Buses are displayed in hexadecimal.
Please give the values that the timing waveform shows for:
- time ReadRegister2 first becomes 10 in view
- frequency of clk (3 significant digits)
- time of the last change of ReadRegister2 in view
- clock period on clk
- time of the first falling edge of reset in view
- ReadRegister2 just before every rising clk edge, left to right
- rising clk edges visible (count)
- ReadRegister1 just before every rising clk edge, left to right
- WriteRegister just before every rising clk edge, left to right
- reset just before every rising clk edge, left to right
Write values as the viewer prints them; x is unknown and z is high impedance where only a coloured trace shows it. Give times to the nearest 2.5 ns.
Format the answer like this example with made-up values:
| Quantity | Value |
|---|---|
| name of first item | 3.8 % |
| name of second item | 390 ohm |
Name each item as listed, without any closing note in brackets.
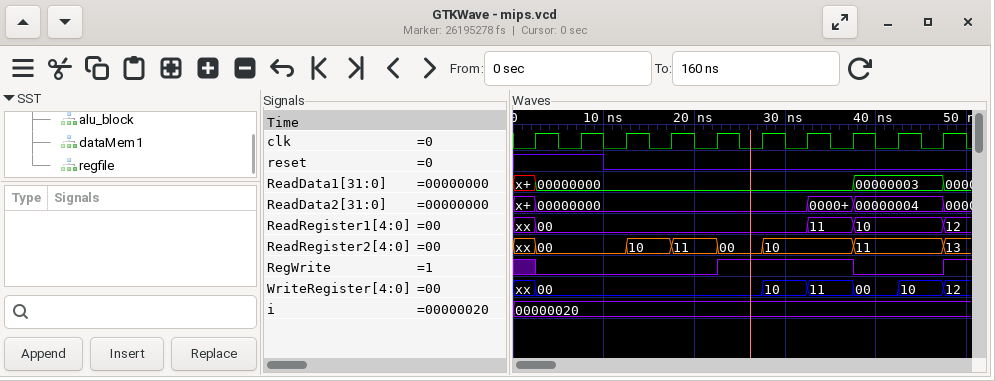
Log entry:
| Quantity | Value |
|---|---|
| time ReadRegister2 first becomes 10 in view | 12.5 ns |
| frequency of clk | 200 MHz |
| time of the last change of ReadRegister2 in view | 47.5 ns |
| clock period on clk | 5 ns |
| time of the first falling edge of reset in view | 10 ns |
| ReadRegister2 just before every rising clk edge, left to right | xx, 00, 00, 10, 11, 00, 10, 10, 11, 11 |
| rising clk edges visible | 10 |
| ReadRegister1 just before every rising clk edge, left to right | xx, 00, 00, 00, 00, 00, 00, 11, 10, 10 |
| WriteRegister just before every rising clk edge, left to right | xx, 00, 00, 00, 00, 00, 10, 11, 00, 10 |
| reset just before every rising clk edge, left to right | 1 1 0 0 0 0 0 0 0 0 |
